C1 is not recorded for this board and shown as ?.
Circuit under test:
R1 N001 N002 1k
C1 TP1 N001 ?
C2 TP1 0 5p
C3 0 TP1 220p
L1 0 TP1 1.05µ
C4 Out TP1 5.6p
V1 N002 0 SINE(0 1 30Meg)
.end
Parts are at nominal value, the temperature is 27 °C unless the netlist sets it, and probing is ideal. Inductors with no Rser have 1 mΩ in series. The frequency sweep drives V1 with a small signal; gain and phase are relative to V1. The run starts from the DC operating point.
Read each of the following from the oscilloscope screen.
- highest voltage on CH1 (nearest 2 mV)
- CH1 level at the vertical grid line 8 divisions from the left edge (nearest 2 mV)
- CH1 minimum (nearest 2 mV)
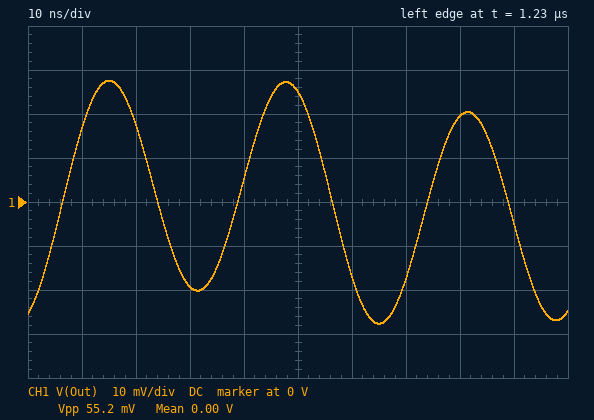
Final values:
28 mV
20 mV
-28 mV
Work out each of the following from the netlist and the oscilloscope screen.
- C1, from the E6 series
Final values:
15 pF
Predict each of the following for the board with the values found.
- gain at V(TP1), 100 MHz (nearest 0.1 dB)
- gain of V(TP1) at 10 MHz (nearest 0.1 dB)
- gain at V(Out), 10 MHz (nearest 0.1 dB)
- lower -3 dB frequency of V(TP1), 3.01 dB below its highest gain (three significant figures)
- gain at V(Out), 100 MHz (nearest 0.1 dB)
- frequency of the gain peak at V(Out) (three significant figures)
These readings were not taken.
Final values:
-43.0 dB
-0.2 dB
-0.2 dB
10.0 MHz
-43.0 dB
10.2 MHz
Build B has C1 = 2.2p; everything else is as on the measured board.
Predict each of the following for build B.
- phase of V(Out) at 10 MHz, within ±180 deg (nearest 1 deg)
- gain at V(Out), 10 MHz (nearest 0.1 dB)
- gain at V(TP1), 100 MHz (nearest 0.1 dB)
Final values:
171 deg
-16.2 dB
-44.8 dB
